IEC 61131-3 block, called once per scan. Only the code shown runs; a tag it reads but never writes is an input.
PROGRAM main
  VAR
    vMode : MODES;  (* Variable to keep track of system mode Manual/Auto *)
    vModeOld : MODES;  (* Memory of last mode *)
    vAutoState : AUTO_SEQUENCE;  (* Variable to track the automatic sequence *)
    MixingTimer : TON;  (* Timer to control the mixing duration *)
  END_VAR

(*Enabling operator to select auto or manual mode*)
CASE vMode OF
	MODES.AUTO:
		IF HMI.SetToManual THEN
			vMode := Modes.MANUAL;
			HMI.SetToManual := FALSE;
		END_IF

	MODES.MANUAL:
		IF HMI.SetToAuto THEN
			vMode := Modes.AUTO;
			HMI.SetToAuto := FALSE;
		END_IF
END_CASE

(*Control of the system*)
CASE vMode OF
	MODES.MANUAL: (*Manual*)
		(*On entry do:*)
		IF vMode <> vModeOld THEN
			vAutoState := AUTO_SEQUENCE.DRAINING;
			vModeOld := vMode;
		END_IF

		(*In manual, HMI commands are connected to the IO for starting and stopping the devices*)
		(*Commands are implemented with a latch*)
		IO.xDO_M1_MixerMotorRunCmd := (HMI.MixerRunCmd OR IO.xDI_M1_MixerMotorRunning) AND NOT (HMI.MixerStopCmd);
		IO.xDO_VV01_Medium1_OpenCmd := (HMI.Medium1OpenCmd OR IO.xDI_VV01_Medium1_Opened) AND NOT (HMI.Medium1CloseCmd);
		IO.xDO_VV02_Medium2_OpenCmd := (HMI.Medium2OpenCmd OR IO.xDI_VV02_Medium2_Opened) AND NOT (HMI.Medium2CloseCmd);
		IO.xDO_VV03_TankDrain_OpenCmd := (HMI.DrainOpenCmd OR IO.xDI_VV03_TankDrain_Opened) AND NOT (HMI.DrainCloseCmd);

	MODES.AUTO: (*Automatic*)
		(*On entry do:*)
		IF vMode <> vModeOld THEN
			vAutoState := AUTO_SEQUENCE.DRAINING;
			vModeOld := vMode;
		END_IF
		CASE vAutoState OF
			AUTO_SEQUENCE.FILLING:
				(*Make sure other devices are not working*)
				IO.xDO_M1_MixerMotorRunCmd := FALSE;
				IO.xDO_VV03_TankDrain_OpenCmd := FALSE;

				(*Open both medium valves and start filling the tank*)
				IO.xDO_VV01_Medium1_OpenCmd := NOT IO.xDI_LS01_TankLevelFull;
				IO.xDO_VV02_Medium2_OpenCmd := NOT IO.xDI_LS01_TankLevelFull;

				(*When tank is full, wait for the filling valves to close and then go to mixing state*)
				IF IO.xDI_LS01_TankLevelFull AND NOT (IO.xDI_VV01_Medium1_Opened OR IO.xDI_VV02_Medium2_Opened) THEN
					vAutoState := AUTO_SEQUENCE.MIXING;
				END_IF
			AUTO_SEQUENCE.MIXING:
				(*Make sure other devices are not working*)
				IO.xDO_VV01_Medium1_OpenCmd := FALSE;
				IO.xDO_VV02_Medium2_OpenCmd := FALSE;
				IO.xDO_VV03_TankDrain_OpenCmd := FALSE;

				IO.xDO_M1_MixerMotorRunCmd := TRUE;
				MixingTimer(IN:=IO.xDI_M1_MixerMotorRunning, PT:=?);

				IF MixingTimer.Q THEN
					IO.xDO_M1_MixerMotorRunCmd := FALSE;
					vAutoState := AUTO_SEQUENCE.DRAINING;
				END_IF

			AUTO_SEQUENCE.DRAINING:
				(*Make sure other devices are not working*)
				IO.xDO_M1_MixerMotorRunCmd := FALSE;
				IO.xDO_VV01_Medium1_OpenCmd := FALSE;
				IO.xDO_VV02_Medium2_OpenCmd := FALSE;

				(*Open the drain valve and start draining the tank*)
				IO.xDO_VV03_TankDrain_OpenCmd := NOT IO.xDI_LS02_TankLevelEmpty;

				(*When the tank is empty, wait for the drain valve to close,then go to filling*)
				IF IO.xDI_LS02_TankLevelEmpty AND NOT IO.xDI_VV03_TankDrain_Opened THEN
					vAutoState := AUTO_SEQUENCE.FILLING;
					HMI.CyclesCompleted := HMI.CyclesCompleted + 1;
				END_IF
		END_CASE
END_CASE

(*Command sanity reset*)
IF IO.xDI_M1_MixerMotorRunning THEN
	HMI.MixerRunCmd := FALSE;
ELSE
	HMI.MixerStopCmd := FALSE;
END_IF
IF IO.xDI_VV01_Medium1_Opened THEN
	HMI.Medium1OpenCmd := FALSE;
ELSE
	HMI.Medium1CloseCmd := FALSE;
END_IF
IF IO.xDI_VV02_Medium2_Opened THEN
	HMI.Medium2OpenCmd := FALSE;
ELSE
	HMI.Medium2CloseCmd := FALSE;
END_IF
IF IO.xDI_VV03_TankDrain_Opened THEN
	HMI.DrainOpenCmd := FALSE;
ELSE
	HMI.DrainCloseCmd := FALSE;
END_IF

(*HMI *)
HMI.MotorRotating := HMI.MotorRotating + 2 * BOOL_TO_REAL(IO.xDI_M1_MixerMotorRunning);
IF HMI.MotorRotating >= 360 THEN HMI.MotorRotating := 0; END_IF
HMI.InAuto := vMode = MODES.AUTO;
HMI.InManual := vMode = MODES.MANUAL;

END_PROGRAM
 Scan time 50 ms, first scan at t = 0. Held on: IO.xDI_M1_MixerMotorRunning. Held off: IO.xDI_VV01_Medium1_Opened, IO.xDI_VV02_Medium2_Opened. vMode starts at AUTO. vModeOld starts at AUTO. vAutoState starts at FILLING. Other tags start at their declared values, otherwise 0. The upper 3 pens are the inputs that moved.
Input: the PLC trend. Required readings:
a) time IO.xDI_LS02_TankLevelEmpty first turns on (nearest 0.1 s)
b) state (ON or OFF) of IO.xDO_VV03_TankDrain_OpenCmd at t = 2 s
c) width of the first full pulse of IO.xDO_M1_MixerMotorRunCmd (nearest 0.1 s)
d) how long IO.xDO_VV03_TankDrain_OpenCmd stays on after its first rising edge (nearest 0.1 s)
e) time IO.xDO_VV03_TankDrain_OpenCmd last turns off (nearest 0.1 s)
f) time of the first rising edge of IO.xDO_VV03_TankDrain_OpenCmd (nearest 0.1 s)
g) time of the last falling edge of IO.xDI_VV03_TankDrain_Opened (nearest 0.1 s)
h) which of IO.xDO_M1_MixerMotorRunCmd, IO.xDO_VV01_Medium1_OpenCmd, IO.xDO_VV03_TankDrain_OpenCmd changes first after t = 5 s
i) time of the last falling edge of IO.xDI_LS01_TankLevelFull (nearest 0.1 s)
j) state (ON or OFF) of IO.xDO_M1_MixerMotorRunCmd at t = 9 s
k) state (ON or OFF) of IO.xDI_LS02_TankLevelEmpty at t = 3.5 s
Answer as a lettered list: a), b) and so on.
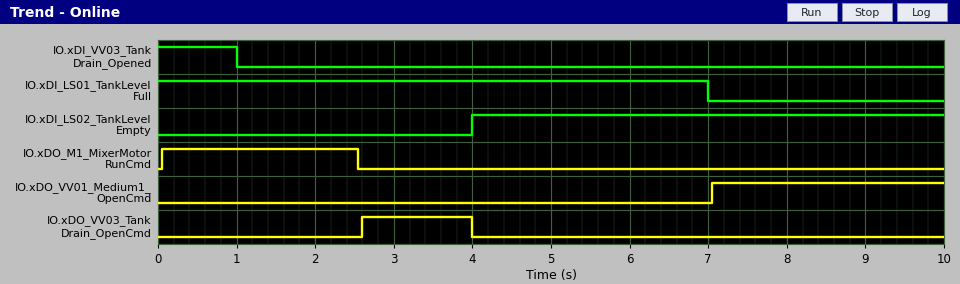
a) 4.0 s
b) OFF
c) 2.5 s
d) 1.4 s
e) 4.0 s
f) 2.6 s
g) 1.0 s
h) IO.xDO_VV01_Medium1_OpenCmd
i) 7.0 s
j) OFF
k) OFF
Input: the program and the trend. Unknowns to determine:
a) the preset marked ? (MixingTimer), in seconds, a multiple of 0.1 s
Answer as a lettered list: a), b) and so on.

a) 2.5 s
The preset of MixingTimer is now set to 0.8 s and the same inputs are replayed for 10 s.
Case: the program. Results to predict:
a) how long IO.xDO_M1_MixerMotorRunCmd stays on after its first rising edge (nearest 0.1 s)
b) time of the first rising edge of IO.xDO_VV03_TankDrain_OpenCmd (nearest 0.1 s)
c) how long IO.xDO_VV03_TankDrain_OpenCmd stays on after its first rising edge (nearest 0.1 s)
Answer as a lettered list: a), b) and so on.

a) 0.8 s
b) 0.9 s
c) 3.1 s
